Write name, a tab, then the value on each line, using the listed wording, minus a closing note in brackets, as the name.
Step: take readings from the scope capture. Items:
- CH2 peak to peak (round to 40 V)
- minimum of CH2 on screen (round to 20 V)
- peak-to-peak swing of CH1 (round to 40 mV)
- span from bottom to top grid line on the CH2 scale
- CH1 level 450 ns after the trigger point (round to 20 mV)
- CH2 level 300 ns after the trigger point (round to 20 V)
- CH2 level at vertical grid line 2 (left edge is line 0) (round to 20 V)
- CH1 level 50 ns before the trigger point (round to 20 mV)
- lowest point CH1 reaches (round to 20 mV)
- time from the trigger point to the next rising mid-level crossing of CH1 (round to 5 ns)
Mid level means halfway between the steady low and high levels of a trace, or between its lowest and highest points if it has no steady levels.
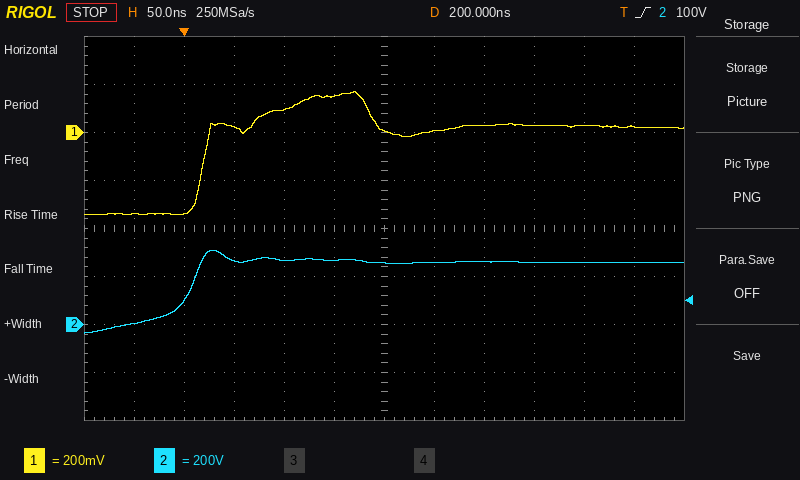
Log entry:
CH2 peak to peak	360 V
minimum of CH2 on screen	-40 V
peak-to-peak swing of CH1	520 mV
span from bottom to top grid line on the CH2 scale	1.6 kV
CH1 level 450 ns after the trigger point	20 mV
CH2 level 300 ns after the trigger point	260 V
CH2 level at vertical grid line 2 (left edge is line 0)	100 V
CH1 level 50 ns before the trigger point	-340 mV
lowest point CH1 reaches	-340 mV
time from the trigger point to the next rising mid-level crossing of CH1	20 ns
